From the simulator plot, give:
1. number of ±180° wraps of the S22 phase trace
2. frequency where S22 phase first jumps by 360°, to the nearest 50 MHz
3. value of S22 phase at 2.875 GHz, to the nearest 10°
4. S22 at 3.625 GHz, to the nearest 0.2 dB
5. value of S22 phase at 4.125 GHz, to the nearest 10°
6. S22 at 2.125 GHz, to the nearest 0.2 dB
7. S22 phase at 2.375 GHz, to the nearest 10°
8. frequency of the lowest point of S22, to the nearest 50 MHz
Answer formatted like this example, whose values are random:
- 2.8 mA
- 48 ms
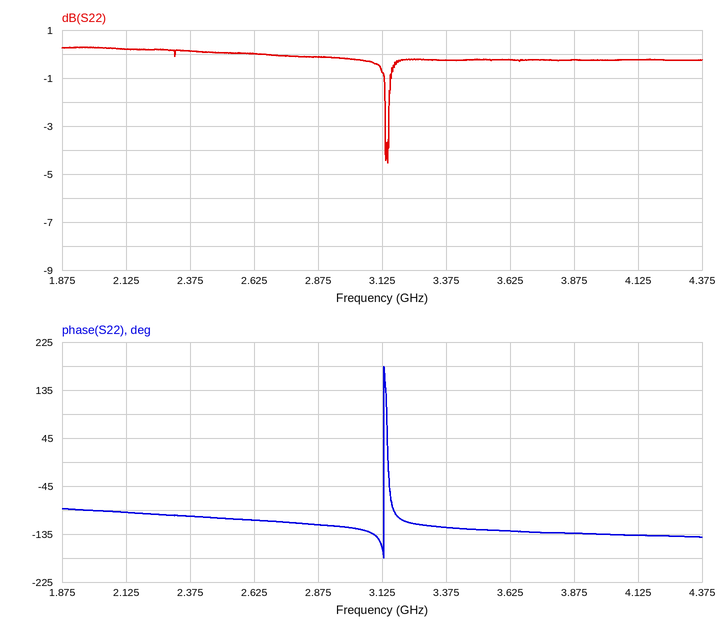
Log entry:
- 1
- 3.15 GHz
- -120°
- -0.2 dB
- -140°
- 0.2 dB
- -100°
- 3.15 GHz
